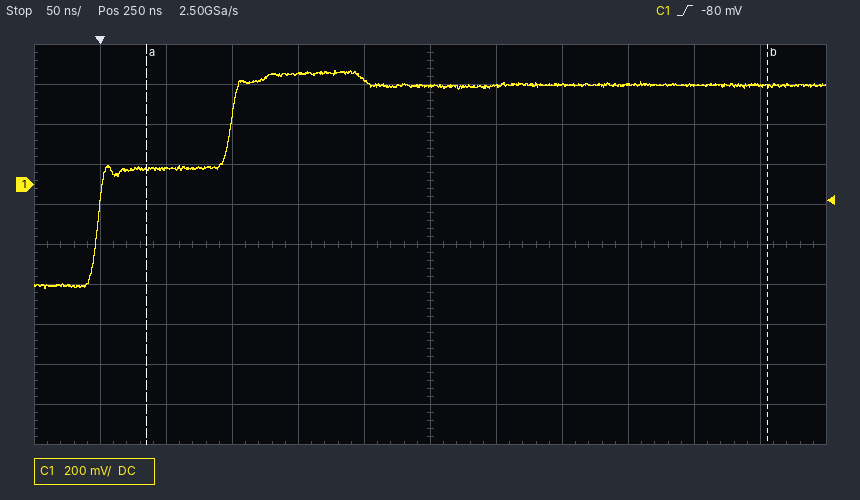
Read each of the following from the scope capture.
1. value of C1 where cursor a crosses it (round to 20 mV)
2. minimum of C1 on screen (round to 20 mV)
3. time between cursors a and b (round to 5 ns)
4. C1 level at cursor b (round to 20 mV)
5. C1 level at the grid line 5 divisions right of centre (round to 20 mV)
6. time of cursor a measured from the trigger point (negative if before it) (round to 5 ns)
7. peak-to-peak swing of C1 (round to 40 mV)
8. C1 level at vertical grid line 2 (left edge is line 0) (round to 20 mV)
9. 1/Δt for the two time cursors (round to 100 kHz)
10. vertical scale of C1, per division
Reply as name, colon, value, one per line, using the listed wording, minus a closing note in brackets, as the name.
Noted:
value of C1 where cursor a crosses it: 80 mV
minimum of C1 on screen: -520 mV
time between cursors a and b: 470 ns
C1 level at cursor b: 500 mV
C1 level at the grid line 5 divisions right of centre: 500 mV
time of cursor a measured from the trigger point (negative if before it): +35 ns
peak-to-peak swing of C1: 1.08 V
C1 level at vertical grid line 2 (left edge is line 0): 80 mV
1/Δt for the two time cursors: 2.1 MHz
vertical scale of C1, per division: 200 mV
